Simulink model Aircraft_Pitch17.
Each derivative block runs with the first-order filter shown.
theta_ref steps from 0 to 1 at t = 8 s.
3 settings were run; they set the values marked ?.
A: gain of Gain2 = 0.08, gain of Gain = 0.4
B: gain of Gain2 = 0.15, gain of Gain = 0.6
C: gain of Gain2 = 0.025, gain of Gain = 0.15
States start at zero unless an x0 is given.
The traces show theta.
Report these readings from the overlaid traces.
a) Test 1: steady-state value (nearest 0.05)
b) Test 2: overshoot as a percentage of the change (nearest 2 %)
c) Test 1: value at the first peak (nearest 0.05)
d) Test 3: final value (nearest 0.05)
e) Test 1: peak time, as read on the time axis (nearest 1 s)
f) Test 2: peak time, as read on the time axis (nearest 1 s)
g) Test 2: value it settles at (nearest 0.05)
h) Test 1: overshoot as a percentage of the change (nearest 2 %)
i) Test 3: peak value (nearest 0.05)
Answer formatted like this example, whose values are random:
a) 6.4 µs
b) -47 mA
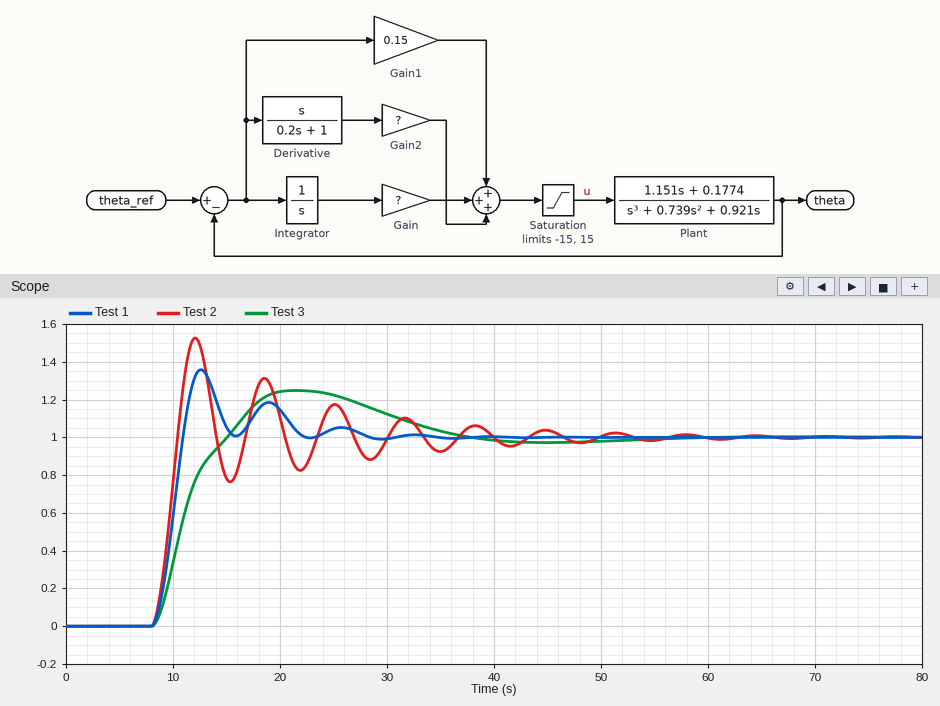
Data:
a) 1.00
b) 52 %
c) 1.35
d) 1.00
e) 13 s
f) 12 s
g) 1.00
h) 36 %
i) 1.25
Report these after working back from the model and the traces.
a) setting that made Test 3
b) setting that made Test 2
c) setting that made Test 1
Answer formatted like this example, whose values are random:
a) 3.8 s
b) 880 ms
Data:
a) C
b) B
c) A
